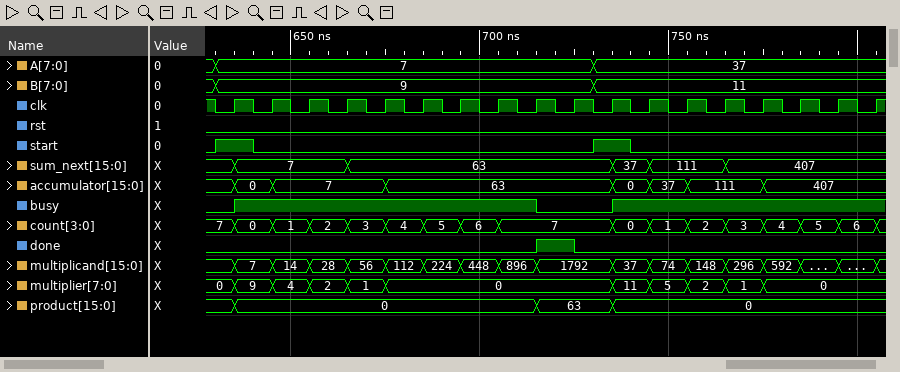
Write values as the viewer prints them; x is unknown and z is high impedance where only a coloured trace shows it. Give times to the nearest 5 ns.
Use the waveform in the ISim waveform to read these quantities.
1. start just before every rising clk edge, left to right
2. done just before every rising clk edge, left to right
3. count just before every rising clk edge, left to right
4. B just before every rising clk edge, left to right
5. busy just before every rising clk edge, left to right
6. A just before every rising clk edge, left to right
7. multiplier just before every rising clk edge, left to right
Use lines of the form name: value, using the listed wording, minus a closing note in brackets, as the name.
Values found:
start just before every rising clk edge, left to right: 1 0 0 0 0 0 0 0 0 0 1 0 0 0 0 0 0 0
done just before every rising clk edge, left to right: 0 0 0 0 0 0 0 0 0 1 0 0 0 0 0 0 0 0
count just before every rising clk edge, left to right: 7, 0, 1, 2, 3, 4, 5, 6, 7, 7, 7, 0, 1, 2, 3, 4, 5, 6
B just before every rising clk edge, left to right: 9, 9, 9, 9, 9, 9, 9, 9, 9, 9, 11, 11, 11, 11, 11, 11, 11, 11
busy just before every rising clk edge, left to right: 0 1 1 1 1 1 1 1 1 0 0 1 1 1 1 1 1 1
A just before every rising clk edge, left to right: 7, 7, 7, 7, 7, 7, 7, 7, 7, 7, 37, 37, 37, 37, 37, 37, 37, 37
multiplier just before every rising clk edge, left to right: 0, 9, 4, 2, 1, 0, 0, 0, 0, 0, 0, 11, 5, 2, 1, 0, 0, 0
